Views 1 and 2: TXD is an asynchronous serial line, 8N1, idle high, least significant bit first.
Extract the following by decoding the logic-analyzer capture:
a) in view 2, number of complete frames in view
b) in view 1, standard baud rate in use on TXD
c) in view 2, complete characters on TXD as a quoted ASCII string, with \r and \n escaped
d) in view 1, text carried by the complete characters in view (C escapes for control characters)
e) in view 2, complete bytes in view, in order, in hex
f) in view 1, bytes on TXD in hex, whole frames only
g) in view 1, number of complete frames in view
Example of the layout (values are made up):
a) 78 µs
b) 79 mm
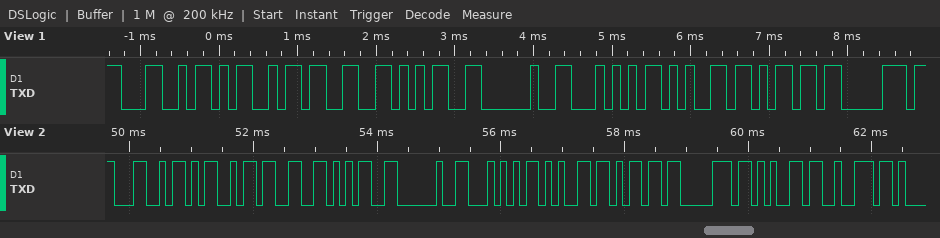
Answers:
a) 11
b) 9600 baud
c) "LM35 Temper"
d) "LM35 Temp"
e) 0x4C 0x4D 0x33 0x35 0x20 0x54 0x65 0x6D 0x70 0x65 0x72
f) 4C 4D 33 35 20 54 65 6D 70
g) 9
